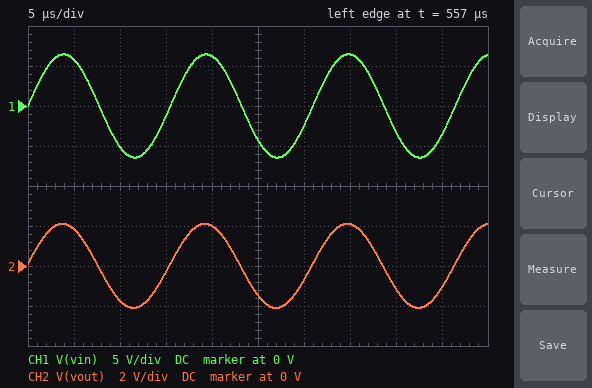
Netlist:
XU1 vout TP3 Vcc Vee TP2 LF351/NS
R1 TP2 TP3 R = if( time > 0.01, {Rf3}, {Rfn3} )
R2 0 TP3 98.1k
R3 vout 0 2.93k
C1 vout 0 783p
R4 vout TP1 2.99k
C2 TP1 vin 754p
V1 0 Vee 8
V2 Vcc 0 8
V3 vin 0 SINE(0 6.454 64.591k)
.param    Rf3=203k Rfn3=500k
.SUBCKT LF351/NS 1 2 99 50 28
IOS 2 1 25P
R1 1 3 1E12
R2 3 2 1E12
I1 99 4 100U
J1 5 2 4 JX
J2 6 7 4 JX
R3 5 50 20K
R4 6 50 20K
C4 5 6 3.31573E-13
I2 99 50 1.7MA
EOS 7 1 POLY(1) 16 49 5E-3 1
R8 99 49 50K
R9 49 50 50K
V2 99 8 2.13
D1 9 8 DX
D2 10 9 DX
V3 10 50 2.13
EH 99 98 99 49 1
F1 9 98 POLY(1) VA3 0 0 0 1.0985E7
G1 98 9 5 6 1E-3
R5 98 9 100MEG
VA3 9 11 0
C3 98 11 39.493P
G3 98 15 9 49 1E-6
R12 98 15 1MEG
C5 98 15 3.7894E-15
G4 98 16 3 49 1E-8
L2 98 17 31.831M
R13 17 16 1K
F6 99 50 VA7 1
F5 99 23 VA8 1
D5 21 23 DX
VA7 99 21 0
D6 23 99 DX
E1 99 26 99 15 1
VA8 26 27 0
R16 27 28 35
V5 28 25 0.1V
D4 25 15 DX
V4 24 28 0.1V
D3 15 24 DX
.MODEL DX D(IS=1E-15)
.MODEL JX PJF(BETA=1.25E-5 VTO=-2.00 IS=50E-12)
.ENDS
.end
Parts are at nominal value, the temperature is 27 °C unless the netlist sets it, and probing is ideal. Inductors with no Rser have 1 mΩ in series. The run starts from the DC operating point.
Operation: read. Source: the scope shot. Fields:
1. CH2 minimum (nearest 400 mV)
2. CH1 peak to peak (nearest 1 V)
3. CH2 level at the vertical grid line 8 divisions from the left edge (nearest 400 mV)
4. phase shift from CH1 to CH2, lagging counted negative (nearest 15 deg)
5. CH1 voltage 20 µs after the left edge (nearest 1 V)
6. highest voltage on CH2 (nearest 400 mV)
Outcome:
-2.0 V
13 V
-1.2 V
0 deg
6 V
2.0 V
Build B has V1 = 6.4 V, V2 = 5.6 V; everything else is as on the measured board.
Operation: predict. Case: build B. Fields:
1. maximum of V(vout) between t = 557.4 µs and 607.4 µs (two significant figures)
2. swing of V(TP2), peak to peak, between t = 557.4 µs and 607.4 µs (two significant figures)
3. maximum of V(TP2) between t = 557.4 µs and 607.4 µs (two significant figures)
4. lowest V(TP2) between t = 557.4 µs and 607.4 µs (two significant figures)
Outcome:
2.1 V
9.2 V
4.2 V
-5.0 V
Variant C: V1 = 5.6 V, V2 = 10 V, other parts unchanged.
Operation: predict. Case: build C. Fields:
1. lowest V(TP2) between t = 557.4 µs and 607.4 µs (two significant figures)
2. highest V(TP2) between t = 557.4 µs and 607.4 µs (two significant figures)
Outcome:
-4.2 V
8.6 V
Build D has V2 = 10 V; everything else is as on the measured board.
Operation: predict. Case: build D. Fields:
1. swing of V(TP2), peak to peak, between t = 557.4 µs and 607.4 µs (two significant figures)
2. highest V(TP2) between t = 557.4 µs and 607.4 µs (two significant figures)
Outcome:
15 V
8.6 V
